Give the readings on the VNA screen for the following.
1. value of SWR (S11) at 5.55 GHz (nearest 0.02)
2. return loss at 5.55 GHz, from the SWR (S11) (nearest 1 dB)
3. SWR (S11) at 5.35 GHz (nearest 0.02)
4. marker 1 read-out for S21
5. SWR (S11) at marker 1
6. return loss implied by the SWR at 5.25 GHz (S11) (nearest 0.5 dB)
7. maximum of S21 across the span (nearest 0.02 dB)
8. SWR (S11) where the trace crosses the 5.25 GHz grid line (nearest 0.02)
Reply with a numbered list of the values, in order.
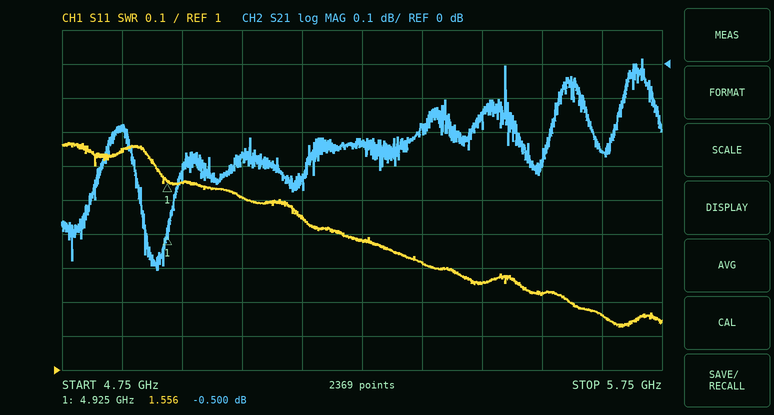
1. 1.22
2. 20 dB
3. 1.32
4. -0.500 dB
5. 1.556
6. 16.0 dB
7. 0.02 dB
8. 1.38
